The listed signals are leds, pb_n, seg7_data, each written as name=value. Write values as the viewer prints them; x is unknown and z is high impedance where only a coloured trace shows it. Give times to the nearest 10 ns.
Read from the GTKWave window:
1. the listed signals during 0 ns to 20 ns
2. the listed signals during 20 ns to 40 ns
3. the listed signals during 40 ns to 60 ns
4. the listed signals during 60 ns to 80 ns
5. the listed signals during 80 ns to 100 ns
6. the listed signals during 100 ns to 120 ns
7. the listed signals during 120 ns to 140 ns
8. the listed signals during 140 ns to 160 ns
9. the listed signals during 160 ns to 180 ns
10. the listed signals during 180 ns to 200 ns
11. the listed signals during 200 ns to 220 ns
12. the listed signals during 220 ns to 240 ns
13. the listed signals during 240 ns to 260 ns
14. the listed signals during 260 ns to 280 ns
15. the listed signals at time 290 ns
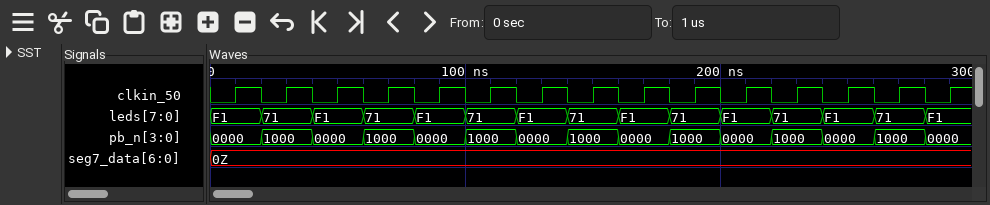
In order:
leds=F1, pb_n=0000, seg7_data=0Z
leds=71, pb_n=1000, seg7_data=0Z
leds=F1, pb_n=0000, seg7_data=0Z
leds=71, pb_n=1000, seg7_data=0Z
leds=F1, pb_n=0000, seg7_data=0Z
leds=71, pb_n=1000, seg7_data=0Z
leds=F1, pb_n=0000, seg7_data=0Z
leds=71, pb_n=1000, seg7_data=0Z
leds=F1, pb_n=0000, seg7_data=0Z
leds=71, pb_n=1000, seg7_data=0Z
leds=F1, pb_n=0000, seg7_data=0Z
leds=71, pb_n=1000, seg7_data=0Z
leds=F1, pb_n=0000, seg7_data=0Z
leds=71, pb_n=1000, seg7_data=0Z
leds=F1, pb_n=0000, seg7_data=0Z
